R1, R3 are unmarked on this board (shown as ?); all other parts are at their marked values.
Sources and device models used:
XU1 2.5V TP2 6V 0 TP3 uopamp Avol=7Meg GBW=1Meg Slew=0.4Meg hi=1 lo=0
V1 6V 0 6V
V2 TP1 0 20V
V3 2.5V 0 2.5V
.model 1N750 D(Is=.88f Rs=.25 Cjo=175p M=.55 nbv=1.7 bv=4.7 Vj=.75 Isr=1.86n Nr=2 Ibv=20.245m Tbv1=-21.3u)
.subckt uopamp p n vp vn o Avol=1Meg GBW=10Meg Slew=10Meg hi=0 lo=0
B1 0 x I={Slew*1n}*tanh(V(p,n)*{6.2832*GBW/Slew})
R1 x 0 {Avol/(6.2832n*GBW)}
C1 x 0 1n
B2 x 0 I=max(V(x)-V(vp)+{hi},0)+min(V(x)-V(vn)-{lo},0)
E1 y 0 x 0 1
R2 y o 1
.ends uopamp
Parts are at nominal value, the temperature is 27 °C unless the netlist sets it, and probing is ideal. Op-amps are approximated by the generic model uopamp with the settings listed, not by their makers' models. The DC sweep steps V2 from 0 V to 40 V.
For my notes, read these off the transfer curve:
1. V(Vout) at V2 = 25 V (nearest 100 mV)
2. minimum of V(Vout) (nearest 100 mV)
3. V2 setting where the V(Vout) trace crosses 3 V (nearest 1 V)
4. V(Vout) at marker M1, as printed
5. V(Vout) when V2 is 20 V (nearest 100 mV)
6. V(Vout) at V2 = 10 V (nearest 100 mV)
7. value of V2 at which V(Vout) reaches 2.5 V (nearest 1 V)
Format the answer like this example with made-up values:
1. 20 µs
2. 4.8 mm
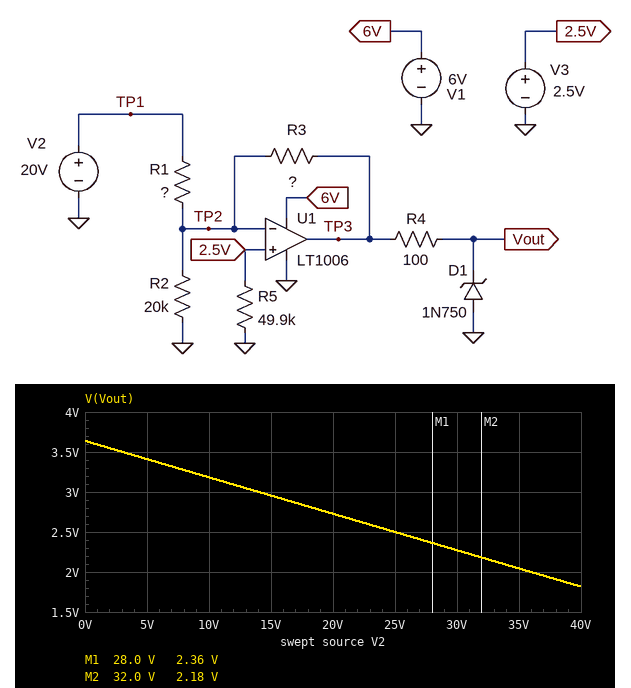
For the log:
1. 2.5 V
2. 1.8 V
3. 14 V
4. 2.36 V
5. 2.7 V
6. 3.2 V
7. 25 V
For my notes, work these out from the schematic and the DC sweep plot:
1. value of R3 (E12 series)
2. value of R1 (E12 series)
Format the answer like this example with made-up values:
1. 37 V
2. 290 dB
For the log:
1. 8.2 kΩ
2. 180 kΩ
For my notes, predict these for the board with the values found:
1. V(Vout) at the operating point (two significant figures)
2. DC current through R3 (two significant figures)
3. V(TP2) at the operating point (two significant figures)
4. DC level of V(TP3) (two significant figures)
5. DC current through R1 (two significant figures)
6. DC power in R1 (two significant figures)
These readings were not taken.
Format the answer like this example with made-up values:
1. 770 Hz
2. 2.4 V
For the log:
1. 2.7 V
2. 28 µA
3. 2.5 V
4. 2.7 V
5. 97 µA
6. 1.7 mW
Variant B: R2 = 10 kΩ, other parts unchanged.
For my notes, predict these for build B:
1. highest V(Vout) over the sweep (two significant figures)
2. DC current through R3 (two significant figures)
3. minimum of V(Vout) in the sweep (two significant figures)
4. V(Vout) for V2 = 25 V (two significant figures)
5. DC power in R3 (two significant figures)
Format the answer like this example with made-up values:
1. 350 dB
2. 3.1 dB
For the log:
1. 4.6 V
2. 150 µA
3. 2.8 V
4. 3.5 V
5. 190 µW
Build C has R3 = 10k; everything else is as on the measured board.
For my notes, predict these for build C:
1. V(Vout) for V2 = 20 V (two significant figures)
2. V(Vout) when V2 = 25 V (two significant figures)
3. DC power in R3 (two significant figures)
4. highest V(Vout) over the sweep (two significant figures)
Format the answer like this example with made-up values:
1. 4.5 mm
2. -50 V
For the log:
1. 2.8 V
2. 2.5 V
3. 7.7 µW
4. 3.9 V
